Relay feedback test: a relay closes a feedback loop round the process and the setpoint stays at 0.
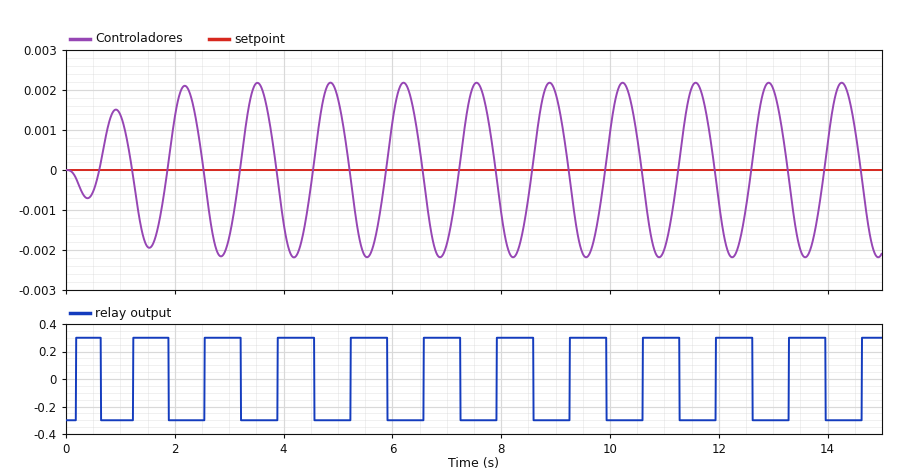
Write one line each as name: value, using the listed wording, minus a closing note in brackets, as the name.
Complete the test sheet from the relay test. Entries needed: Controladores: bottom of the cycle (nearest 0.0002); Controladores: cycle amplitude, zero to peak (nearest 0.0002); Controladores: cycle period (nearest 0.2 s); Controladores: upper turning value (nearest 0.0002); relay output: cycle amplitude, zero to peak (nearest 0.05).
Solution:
Controladores: bottom of the cycle: -0.0022
Controladores: cycle amplitude, zero to peak: 0.0022
Controladores: cycle period: 1.4 s
Controladores: upper turning value: 0.0022
relay output: cycle amplitude, zero to peak: 0.30
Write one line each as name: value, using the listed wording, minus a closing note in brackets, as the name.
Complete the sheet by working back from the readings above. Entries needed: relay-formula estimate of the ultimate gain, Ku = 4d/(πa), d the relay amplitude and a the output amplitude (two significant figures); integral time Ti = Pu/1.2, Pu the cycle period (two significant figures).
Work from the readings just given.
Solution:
relay-formula estimate of the ultimate gain, Ku = 4d/(πa), d the relay amplitude and a the output amplitude: 170
integral time Ti = Pu/1.2, Pu the cycle period: 1.2 s
